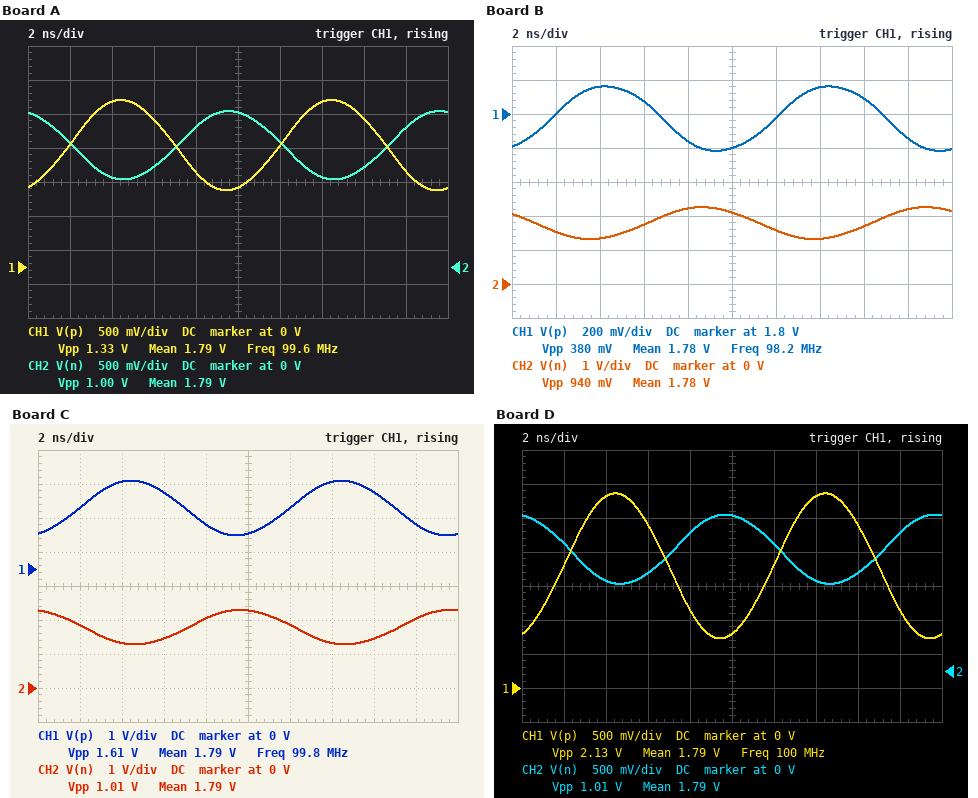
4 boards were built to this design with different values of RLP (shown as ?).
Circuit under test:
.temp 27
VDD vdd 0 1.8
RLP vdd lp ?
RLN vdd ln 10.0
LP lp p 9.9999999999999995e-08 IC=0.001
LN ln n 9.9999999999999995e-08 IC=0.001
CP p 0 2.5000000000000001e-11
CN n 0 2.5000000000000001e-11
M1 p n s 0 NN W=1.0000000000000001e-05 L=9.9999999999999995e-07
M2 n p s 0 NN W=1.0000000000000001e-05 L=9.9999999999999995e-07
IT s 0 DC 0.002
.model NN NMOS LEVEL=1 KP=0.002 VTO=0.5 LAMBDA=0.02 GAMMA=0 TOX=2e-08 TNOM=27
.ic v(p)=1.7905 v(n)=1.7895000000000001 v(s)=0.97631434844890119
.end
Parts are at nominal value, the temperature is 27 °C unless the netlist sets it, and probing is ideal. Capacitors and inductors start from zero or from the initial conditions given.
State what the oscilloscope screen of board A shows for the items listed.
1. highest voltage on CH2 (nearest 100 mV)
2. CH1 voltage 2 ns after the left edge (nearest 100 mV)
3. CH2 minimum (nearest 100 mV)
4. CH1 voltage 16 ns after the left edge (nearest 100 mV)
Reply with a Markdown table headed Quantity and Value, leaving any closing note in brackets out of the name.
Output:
| Quantity | Value |
|---|---|
| highest voltage on CH2 | 2.3 V |
| CH1 voltage 2 ns after the left edge | 1.8 V |
| CH2 minimum | 1.3 V |
| CH1 voltage 16 ns after the left edge | 2.2 V |
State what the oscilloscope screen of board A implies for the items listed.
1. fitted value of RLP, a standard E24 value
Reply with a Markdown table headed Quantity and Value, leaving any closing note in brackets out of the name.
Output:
| Quantity | Value |
|---|---|
| fitted value of RLP, a standard E24 value | 7.5 Ω |
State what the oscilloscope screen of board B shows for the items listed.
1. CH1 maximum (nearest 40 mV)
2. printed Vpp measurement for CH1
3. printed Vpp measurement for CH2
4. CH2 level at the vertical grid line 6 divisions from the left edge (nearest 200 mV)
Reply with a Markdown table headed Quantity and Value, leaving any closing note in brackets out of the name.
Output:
| Quantity | Value |
|---|---|
| CH1 maximum | 1.96 V |
| printed Vpp measurement for CH1 | 380 mV |
| printed Vpp measurement for CH2 | 940 mV |
| CH2 level at the vertical grid line 6 divisions from the left edge | 1.6 V |
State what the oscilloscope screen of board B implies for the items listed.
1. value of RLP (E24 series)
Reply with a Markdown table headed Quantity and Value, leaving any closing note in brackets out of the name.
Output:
| Quantity | Value |
|---|---|
| value of RLP | 27 Ω |
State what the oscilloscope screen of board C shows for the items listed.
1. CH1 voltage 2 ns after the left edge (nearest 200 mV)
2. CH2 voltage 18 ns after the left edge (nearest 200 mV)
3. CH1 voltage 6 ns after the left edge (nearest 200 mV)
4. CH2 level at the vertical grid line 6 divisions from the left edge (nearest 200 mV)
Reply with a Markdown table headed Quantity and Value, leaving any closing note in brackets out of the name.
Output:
| Quantity | Value |
|---|---|
| CH1 voltage 2 ns after the left edge | 1.8 V |
| CH2 voltage 18 ns after the left edge | 2.0 V |
| CH1 voltage 6 ns after the left edge | 2.2 V |
| CH2 level at the vertical grid line 6 divisions from the left edge | 1.8 V |
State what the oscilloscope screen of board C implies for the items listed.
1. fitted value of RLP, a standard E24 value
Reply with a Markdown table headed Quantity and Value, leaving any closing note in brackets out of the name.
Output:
| Quantity | Value |
|---|---|
| fitted value of RLP, a standard E24 value | 6.2 Ω |
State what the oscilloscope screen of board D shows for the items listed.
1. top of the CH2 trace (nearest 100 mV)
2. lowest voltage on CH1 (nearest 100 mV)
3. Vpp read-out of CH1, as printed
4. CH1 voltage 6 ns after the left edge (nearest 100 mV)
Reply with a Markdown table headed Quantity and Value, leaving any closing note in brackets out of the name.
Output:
| Quantity | Value |
|---|---|
| top of the CH2 trace | 2.3 V |
| lowest voltage on CH1 | 700 mV |
| Vpp read-out of CH1, as printed | 2.13 V |
| CH1 voltage 6 ns after the left edge | 2.4 V |
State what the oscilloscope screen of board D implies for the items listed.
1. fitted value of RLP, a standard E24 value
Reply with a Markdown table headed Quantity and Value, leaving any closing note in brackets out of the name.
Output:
| Quantity | Value |
|---|---|
| fitted value of RLP, a standard E24 value | 4.7 Ω |
